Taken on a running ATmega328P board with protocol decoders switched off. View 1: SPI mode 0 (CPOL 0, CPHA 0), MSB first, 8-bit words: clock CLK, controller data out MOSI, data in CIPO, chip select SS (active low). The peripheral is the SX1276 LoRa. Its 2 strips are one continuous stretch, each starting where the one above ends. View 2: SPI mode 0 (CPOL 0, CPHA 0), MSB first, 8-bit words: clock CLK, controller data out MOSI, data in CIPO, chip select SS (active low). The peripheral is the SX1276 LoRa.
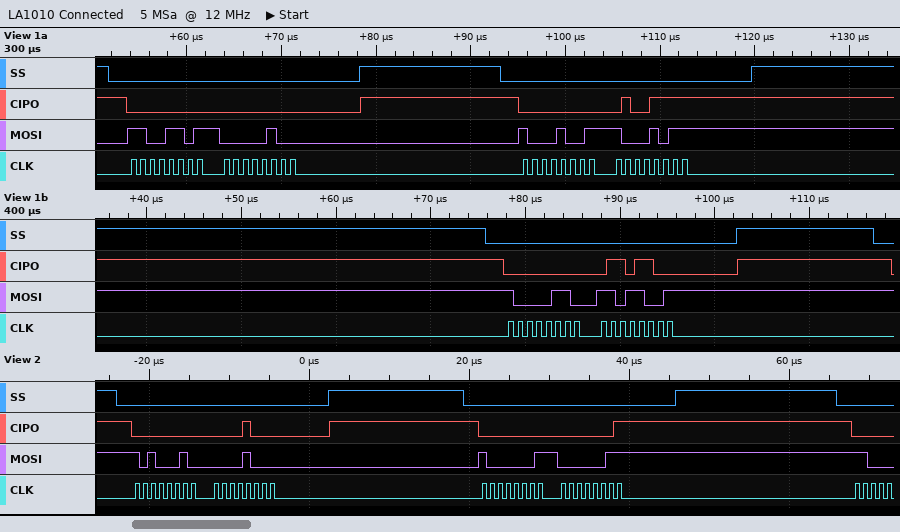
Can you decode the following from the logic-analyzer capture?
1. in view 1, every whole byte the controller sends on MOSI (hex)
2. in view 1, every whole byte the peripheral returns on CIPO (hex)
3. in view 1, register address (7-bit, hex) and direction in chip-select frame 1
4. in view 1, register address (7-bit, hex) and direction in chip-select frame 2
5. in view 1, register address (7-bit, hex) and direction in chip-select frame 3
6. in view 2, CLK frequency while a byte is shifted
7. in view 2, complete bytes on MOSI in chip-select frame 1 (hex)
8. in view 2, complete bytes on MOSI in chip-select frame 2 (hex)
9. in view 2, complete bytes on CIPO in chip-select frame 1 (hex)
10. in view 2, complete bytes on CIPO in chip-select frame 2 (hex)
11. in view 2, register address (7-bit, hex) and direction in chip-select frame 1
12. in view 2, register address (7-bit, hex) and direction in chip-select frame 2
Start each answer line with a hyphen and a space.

- 0xCD 0x04 0x89 0x8B 0x86 0xD9
- 0x00 0x00 0x00 0x4F 0x00 0x6C
- 0x4D write
- 0x09 write
- 0x06 write
- 1 MHz
- A2 08
- 81 03
- 00 08
- 00 01
- 0x22 write
- 0x01 write
